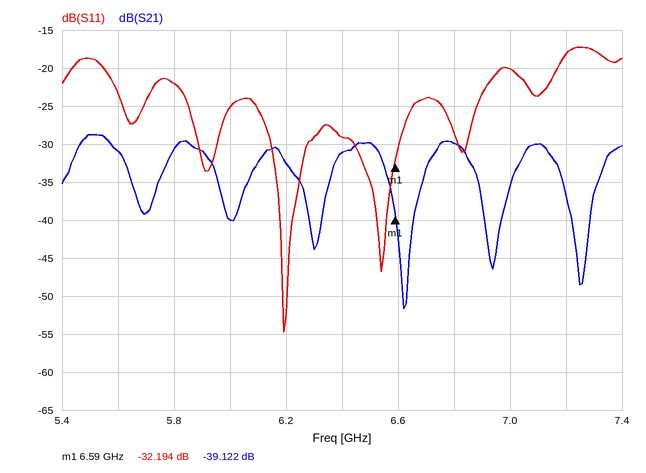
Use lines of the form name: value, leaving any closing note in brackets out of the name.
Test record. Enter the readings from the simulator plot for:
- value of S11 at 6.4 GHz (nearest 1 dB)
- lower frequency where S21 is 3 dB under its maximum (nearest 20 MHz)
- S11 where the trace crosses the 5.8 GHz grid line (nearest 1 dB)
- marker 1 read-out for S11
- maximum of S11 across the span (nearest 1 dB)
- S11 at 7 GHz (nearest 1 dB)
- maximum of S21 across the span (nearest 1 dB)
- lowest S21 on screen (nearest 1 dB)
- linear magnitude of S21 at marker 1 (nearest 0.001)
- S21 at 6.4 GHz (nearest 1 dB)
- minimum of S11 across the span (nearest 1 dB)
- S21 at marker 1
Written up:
value of S11 at 6.4 GHz: -29 dB
lower frequency where S21 is 3 dB under its maximum: 5.44 GHz
S11 where the trace crosses the 5.8 GHz grid line: -22 dB
marker 1 read-out for S11: -32.194 dB
maximum of S11 across the span: -17 dB
S11 at 7 GHz: -20 dB
maximum of S21 across the span: -29 dB
lowest S21 on screen: -52 dB
linear magnitude of S21 at marker 1: 0.011
S21 at 6.4 GHz: -31 dB
minimum of S11 across the span: -55 dB
S21 at marker 1: -39.122 dB
